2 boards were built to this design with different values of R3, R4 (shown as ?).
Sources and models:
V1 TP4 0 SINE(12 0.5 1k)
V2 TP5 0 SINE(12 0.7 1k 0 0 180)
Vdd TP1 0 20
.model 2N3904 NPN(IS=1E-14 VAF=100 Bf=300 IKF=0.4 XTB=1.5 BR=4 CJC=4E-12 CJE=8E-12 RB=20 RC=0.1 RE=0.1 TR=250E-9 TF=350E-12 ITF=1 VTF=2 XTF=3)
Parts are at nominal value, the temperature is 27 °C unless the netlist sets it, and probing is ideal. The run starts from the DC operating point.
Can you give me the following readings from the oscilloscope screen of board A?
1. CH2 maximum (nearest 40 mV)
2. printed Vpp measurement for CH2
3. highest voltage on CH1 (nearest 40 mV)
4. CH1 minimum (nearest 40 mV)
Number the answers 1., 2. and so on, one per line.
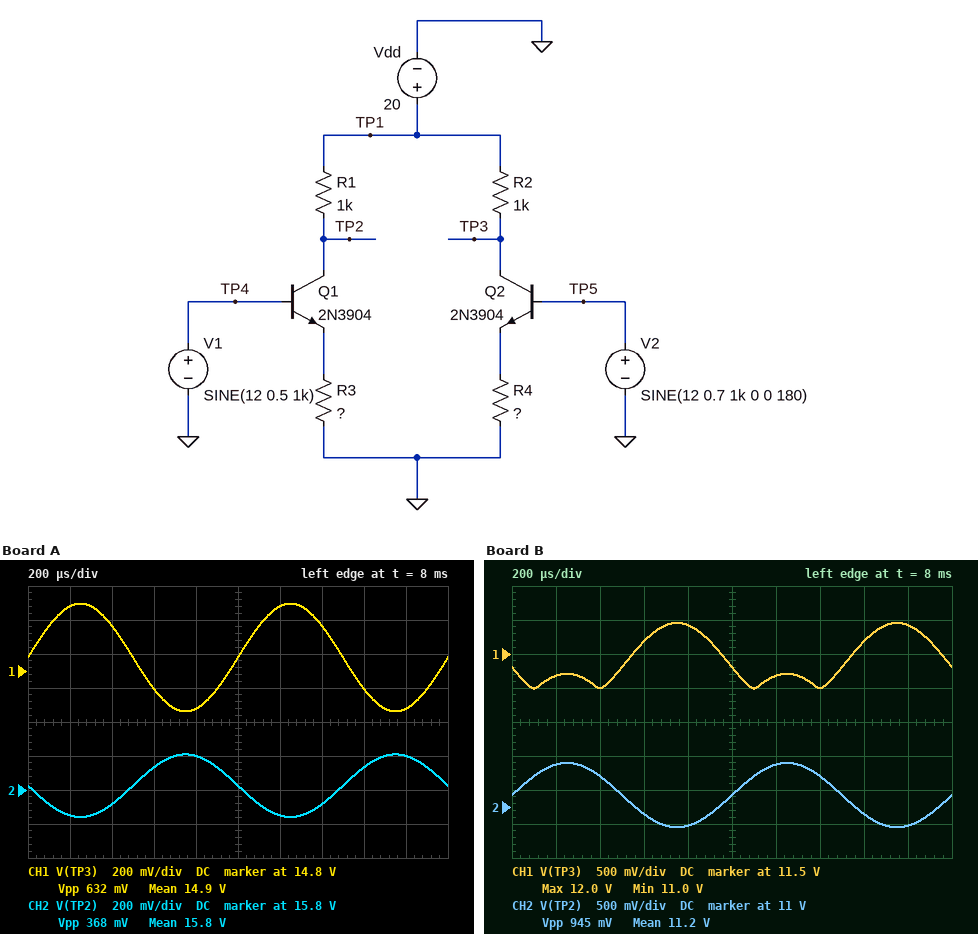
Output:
1. 16.00 V
2. 368 mV
3. 15.20 V
4. 14.56 V
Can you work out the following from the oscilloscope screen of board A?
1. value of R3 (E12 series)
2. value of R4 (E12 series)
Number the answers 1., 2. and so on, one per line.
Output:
1. 2.7 kΩ
2. 2.2 kΩ
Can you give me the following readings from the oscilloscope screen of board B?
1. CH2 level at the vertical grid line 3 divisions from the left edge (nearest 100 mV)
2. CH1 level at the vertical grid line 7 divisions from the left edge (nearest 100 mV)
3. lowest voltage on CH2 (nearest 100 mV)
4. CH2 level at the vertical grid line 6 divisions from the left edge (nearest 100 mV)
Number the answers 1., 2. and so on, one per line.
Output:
1. 10.9 V
2. 11.0 V
3. 10.7 V
4. 11.6 V
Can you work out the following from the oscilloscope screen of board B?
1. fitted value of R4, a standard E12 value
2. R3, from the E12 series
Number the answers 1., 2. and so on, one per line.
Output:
1. 1.2 kΩ
2. 820 Ω
